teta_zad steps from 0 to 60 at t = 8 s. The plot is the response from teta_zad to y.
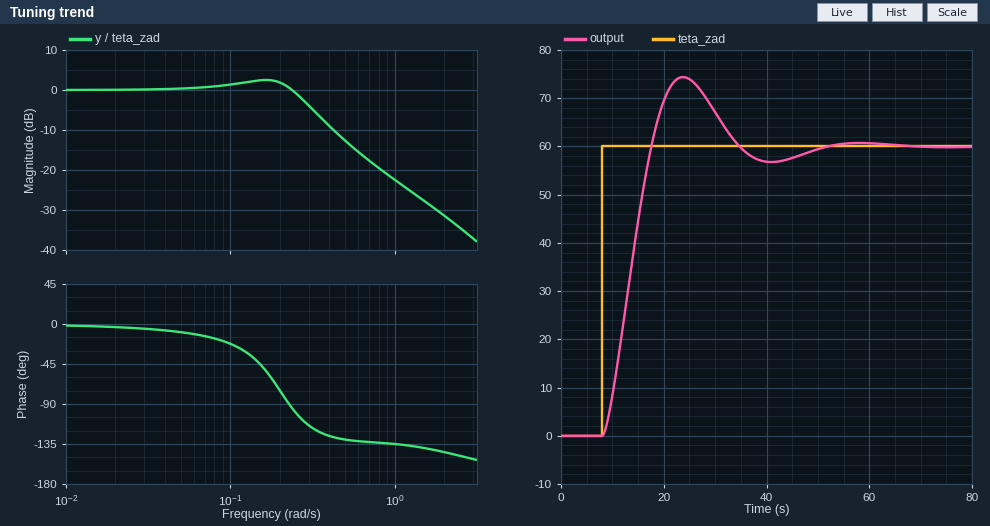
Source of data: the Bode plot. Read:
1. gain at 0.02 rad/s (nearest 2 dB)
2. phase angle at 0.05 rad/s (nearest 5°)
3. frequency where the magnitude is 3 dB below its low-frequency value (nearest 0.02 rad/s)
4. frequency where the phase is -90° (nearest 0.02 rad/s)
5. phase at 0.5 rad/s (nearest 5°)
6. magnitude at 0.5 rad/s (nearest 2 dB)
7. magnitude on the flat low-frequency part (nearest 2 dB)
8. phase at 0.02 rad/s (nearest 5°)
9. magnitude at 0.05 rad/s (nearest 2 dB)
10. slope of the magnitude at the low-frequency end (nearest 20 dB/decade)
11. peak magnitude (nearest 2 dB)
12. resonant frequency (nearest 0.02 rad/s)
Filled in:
0 dB
-10°
0.28 rad/s
0.22 rad/s
-130°
-12 dB
0 dB
-5°
0 dB
0 dB/decade
2 dB
0.16 rad/s
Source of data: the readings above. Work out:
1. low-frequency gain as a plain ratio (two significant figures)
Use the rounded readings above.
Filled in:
1.0
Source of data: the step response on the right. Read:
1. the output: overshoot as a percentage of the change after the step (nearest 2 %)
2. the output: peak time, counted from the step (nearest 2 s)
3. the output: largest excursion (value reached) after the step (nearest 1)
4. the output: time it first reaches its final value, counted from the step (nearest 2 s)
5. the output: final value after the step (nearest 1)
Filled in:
24 %
16 s
74
10 s
60
